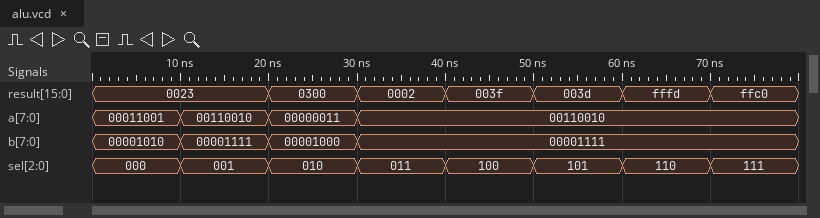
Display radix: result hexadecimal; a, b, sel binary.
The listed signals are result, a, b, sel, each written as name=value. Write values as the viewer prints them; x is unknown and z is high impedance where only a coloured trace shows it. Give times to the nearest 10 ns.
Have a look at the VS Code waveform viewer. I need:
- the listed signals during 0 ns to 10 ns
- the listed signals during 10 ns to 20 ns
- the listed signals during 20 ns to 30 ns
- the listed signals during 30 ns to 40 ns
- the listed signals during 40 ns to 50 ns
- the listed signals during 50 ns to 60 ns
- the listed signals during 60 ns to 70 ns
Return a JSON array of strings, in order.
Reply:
["result=0023, a=00011001, b=00001010, sel=000", "result=0023, a=00110010, b=00001111, sel=001", "result=0300, a=00000011, b=00001000, sel=010", "result=0002, a=00110010, b=00001111, sel=011", "result=003f, a=00110010, b=00001111, sel=100", "result=003d, a=00110010, b=00001111, sel=101", "result=fffd, a=00110010, b=00001111, sel=110"]
